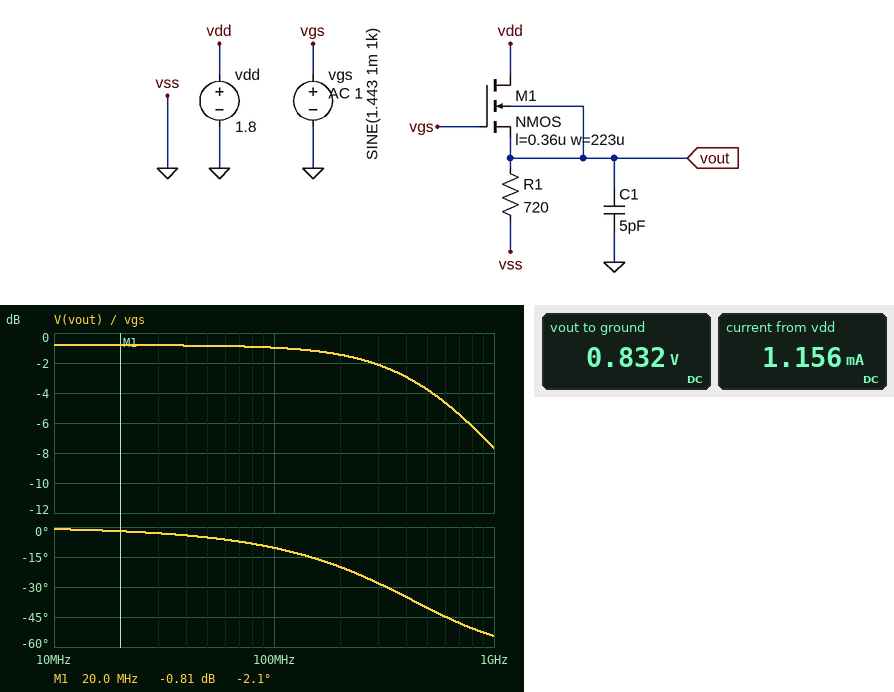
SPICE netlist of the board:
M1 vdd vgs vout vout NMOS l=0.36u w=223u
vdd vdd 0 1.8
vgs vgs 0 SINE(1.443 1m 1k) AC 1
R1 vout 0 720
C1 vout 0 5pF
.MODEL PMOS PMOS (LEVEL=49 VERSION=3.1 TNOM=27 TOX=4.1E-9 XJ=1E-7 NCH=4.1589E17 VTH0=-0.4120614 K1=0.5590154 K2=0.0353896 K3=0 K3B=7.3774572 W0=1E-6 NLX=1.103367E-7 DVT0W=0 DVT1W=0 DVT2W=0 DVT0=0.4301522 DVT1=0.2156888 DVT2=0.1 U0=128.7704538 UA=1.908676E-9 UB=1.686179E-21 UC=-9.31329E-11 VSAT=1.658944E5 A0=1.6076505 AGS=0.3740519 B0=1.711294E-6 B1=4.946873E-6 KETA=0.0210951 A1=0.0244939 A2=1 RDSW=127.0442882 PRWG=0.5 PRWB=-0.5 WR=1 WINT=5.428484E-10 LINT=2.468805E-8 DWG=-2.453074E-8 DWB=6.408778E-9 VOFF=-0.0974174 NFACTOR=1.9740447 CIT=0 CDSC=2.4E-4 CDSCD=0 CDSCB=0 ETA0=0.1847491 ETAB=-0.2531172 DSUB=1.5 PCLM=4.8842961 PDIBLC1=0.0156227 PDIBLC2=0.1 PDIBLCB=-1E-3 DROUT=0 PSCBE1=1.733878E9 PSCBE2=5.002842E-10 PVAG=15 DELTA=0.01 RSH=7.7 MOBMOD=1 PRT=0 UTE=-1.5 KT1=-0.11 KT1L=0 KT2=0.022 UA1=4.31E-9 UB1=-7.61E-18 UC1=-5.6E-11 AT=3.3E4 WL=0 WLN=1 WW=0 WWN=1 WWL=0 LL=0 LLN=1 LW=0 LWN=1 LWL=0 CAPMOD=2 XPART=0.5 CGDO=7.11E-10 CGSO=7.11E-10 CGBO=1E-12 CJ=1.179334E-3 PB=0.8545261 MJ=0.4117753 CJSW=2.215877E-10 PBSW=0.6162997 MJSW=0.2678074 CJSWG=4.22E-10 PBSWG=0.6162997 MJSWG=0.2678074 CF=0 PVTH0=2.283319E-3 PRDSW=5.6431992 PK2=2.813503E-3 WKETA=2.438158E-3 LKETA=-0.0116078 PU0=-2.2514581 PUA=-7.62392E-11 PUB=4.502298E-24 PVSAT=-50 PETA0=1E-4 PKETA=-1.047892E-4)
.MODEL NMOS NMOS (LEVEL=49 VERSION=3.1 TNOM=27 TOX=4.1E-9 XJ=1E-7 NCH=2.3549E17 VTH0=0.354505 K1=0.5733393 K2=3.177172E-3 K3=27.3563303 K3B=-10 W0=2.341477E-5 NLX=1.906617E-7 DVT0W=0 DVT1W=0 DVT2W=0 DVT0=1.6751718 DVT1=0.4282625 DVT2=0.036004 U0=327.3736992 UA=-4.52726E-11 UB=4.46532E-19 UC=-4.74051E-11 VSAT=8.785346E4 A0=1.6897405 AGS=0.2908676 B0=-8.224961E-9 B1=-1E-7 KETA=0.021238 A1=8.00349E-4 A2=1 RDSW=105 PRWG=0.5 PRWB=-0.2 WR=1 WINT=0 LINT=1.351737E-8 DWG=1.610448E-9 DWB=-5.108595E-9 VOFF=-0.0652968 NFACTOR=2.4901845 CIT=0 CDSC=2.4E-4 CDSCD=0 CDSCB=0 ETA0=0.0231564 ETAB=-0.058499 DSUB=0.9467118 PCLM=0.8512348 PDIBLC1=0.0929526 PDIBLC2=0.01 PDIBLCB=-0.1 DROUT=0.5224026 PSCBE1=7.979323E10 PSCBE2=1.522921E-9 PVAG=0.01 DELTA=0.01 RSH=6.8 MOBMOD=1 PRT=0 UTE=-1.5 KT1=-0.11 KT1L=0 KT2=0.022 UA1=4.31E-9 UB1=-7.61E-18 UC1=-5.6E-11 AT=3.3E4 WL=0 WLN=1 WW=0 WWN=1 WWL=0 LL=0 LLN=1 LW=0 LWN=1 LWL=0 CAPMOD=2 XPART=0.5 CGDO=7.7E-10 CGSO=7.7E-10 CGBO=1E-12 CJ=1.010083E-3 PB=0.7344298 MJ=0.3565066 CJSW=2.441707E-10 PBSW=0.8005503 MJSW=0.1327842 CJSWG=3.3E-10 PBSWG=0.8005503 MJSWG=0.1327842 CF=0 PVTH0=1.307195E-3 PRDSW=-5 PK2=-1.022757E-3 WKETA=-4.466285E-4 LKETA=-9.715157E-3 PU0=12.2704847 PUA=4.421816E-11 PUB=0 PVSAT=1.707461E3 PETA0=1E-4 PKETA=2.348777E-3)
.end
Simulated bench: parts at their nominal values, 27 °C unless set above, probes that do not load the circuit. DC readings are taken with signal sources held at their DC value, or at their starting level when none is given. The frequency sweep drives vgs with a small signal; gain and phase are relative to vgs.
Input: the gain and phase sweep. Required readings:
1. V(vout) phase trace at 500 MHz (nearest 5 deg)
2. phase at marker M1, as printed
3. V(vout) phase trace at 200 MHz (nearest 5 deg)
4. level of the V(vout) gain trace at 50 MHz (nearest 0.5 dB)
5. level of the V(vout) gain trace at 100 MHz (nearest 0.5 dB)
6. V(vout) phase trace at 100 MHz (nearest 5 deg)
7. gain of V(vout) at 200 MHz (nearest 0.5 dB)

-40 deg
-2.1 deg
-20 deg
-1.0 dB
-1.0 dB
-10 deg
-1.5 dB
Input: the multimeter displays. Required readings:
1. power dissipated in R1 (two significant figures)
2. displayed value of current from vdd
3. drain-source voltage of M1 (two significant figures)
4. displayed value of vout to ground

960 µW
1.156 mA
970 mV
0.832 V
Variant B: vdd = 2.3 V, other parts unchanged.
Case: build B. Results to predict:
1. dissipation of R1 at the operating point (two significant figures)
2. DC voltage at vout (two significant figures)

970 µW
840 mV
